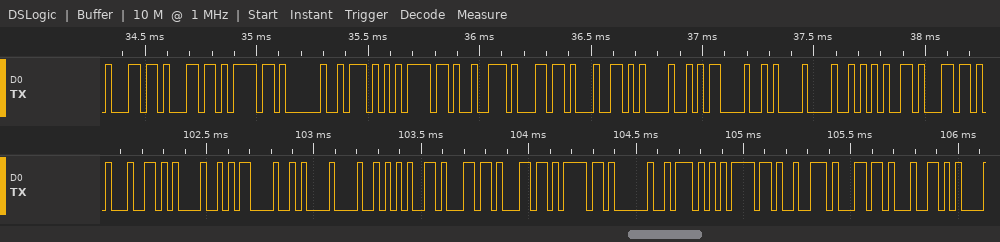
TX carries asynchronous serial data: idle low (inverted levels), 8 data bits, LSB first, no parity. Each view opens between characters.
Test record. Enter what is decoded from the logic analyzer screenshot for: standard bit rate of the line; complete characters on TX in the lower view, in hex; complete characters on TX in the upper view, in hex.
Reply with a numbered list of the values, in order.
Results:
1. 38400 baud
2. 37, BD, E5, EB, 6F, 35, 27, 27, 21, BF, 51, 21, 1B, 27, 37
3. 27, 27, 21, BF, 51, 21, 1B, 27, 37, BD, E5, EB, 6F, 35, 27
